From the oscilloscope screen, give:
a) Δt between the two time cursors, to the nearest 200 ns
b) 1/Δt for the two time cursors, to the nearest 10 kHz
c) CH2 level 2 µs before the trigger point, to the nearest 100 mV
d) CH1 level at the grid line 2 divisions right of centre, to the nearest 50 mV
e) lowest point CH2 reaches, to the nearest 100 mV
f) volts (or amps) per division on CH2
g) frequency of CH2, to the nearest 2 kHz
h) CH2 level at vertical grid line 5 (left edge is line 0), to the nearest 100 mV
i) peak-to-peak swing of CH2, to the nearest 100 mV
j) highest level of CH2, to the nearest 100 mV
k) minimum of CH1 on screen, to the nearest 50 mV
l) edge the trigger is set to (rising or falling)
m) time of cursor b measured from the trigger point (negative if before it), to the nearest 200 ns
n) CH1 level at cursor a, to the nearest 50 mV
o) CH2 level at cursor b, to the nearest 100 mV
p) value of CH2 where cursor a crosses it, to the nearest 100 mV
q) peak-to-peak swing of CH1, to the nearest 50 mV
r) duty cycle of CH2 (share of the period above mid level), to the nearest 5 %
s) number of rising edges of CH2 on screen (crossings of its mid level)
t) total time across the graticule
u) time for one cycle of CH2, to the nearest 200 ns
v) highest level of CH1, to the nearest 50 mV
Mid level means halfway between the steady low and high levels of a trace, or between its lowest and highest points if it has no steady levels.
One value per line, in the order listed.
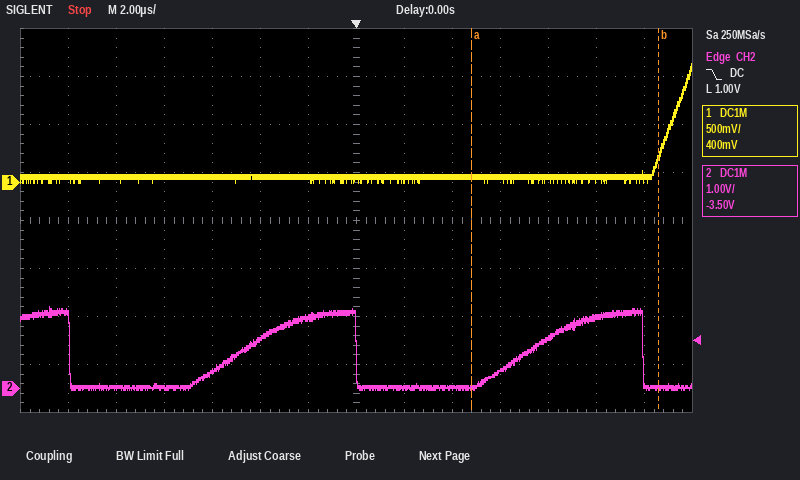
7.8 µs
130 kHz
1.5 V
50 mV
0.0 V
1 V
84 kHz
1.0 V
1.7 V
1.7 V
0 mV
falling
+12.6 µs
50 mV
0.0 V
0.0 V
1.25 V
40 %
2
28 µs
12.0 µs
1.25 V
